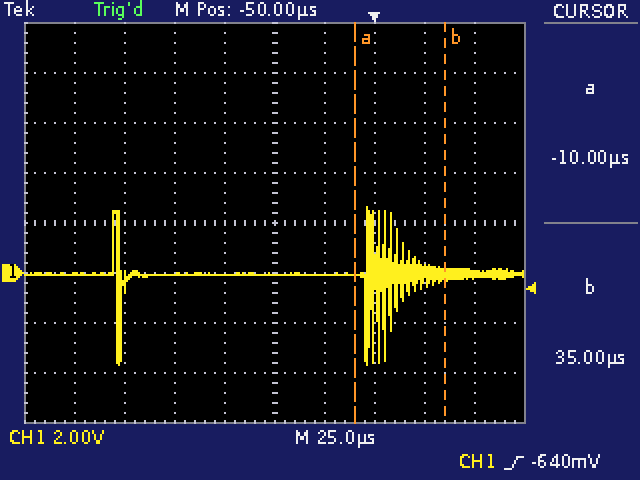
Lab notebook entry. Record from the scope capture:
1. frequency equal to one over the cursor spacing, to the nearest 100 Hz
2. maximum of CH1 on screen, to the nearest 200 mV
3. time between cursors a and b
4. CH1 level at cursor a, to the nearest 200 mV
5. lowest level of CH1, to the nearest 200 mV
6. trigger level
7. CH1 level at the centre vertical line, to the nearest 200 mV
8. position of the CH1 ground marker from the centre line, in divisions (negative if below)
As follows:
22.2 kHz
2.6 V
45.0 µs
0.0 V
-3.6 V
-640 mV
0.0 V
-1.0 div
